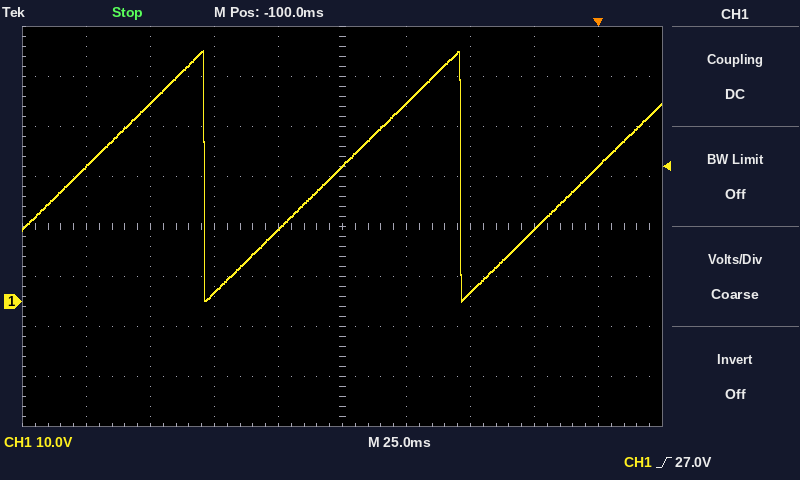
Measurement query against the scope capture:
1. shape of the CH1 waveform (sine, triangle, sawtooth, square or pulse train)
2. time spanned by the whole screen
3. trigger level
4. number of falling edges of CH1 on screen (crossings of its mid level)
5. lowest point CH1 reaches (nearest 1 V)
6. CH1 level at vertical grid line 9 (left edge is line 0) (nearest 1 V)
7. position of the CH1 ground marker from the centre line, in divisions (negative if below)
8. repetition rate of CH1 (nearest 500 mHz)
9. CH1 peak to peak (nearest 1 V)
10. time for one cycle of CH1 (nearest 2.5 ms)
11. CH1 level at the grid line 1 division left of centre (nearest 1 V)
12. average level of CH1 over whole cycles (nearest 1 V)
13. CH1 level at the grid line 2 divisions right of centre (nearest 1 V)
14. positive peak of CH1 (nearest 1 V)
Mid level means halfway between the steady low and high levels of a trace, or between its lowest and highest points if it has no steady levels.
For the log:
sawtooth
250 ms
27.0 V
2
0 V
27 V
-1.5 div
10.0 Hz
50 V
100.0 ms
14 V
25 V
2 V
50 V
